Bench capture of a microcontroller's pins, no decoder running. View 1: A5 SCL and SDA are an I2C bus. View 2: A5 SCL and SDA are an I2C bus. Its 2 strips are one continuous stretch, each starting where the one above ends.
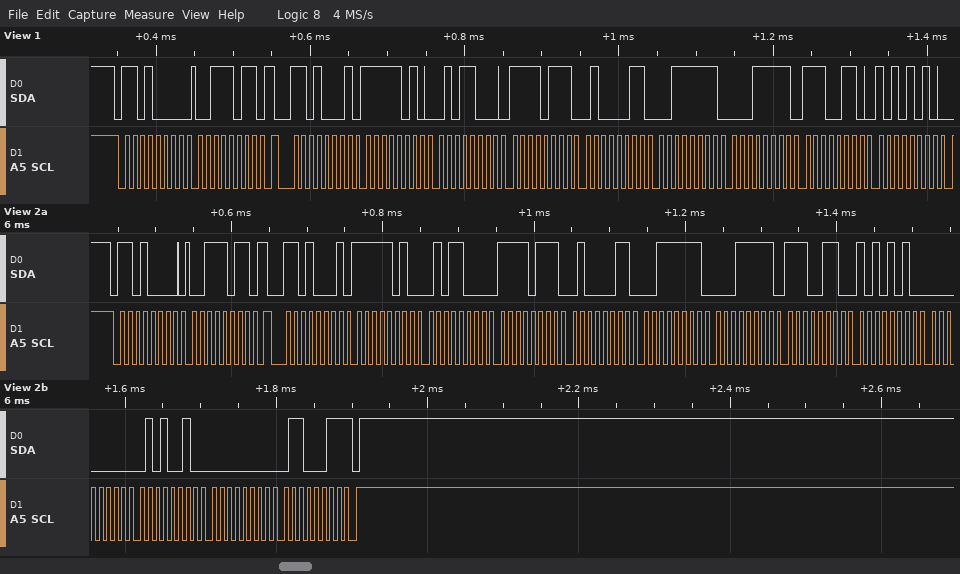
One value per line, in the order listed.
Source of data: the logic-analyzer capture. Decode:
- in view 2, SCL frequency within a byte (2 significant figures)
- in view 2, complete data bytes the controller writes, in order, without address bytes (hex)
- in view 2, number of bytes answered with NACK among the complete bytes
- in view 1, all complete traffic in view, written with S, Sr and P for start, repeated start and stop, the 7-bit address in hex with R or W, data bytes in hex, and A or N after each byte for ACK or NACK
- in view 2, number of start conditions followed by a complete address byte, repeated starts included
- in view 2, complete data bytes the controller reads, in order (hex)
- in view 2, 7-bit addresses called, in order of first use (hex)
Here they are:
100 kHz
3B
1
S 68W A 3B A Sr 68R A FA A 58 A F7 A 43 A 3F A 1F A E6 A AA A
2
FA 58 F7 43 3F 1F E6 AA 00 52 00 63
0x68
